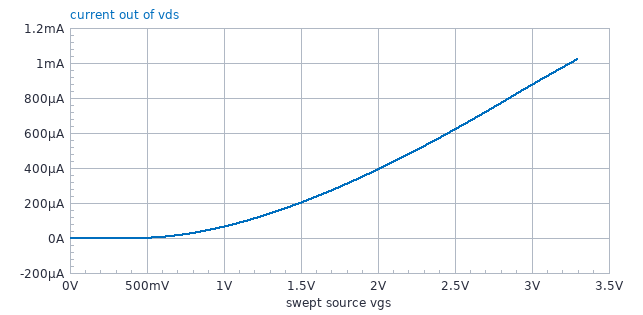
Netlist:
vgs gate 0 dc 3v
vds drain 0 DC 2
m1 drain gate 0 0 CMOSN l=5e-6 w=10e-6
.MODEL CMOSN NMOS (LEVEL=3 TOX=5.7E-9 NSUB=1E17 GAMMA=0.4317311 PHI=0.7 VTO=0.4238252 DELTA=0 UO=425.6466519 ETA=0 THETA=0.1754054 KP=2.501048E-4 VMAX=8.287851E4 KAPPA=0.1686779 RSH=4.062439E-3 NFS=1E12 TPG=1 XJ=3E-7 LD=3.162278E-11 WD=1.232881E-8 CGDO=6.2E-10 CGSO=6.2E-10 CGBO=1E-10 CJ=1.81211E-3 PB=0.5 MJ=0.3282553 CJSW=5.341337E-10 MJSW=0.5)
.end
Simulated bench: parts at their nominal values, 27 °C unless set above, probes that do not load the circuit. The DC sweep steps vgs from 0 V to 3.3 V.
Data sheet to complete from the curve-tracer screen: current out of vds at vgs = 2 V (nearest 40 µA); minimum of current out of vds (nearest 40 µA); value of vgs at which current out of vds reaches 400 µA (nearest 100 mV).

400 µA
0 A
2.0 V
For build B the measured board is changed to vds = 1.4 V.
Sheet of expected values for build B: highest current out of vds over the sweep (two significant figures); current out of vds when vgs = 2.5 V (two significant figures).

890 µA
600 µA
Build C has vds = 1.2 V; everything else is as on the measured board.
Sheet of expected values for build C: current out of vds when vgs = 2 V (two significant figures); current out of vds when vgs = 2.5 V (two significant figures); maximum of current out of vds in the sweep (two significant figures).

390 µA
570 µA
810 µA
